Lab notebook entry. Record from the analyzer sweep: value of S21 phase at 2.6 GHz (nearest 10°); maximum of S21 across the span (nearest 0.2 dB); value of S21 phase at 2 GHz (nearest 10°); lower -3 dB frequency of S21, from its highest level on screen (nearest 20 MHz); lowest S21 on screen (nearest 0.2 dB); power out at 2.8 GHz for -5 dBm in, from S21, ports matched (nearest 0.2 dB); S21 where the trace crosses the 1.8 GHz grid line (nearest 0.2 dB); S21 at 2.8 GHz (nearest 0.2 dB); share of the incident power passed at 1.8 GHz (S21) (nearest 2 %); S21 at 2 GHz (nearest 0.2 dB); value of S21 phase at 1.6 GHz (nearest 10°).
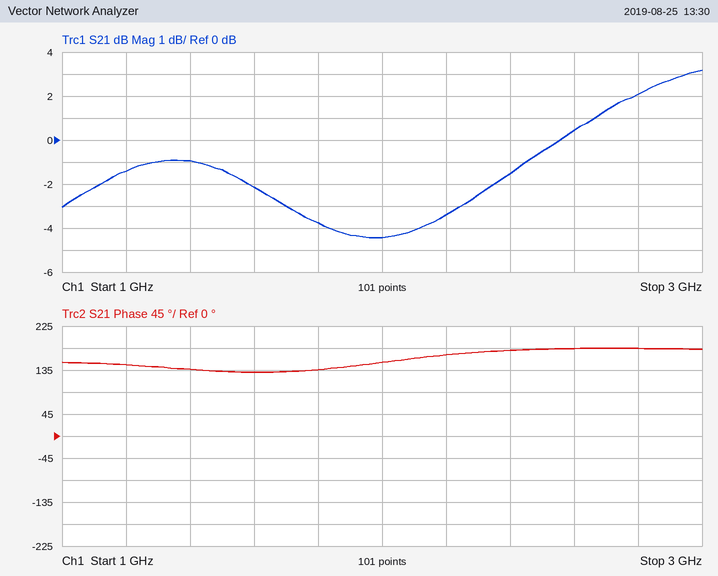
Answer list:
180°
3.2 dB
150°
2.58 GHz
-4.4 dB
-3.0 dBm
-3.8 dB
2.0 dB
42 %
-4.4 dB
130°
